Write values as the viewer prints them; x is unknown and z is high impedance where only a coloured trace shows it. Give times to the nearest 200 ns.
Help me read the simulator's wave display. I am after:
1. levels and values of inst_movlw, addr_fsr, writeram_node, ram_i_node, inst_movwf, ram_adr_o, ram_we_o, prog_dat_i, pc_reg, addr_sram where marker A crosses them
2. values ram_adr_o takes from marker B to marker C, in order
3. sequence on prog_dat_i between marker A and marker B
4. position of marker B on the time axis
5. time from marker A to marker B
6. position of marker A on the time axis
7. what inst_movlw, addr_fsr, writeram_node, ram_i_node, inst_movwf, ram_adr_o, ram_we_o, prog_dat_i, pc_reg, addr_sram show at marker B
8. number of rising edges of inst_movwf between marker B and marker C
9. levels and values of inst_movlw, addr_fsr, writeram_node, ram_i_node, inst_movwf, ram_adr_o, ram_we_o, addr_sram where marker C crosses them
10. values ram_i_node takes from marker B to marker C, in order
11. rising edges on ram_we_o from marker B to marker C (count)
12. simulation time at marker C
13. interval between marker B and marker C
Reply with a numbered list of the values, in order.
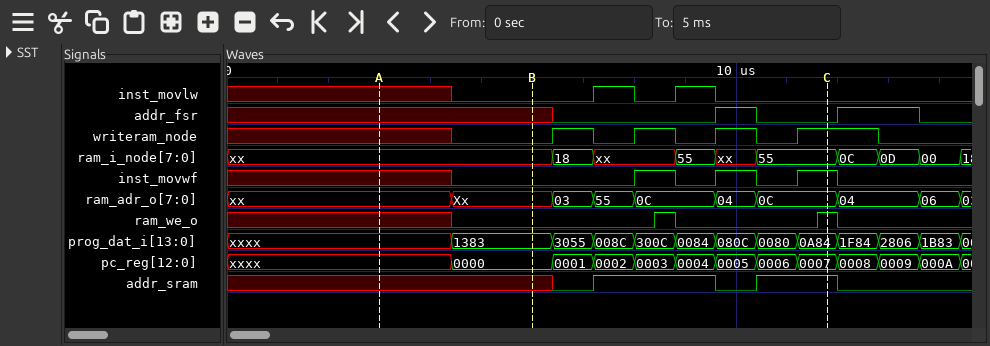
1. inst_movlw=x, addr_fsr=x, writeram_node=x, ram_i_node=xx, inst_movwf=x, ram_adr_o=xx, ram_we_o=x, prog_dat_i=xxxx, pc_reg=xxxx, addr_sram=x
2. Xx, 03, 55, 0C, 04, 0C
3. xxxx, 1383
4. 6000 ns
5. 3000 ns
6. 3000 ns
7. inst_movlw=0, addr_fsr=x, writeram_node=0, ram_i_node=xx, inst_movwf=0, ram_adr_o=Xx, ram_we_o=0, prog_dat_i=1383, pc_reg=0000, addr_sram=x
8. 3
9. inst_movlw=0, addr_fsr=0, writeram_node=1, ram_i_node=55, inst_movwf=1, ram_adr_o=0C, ram_we_o=1, addr_sram=1
10. xx, 18, xx, 55, xx, 55
11. 2
12. 11800 ns
13. 5800 ns
